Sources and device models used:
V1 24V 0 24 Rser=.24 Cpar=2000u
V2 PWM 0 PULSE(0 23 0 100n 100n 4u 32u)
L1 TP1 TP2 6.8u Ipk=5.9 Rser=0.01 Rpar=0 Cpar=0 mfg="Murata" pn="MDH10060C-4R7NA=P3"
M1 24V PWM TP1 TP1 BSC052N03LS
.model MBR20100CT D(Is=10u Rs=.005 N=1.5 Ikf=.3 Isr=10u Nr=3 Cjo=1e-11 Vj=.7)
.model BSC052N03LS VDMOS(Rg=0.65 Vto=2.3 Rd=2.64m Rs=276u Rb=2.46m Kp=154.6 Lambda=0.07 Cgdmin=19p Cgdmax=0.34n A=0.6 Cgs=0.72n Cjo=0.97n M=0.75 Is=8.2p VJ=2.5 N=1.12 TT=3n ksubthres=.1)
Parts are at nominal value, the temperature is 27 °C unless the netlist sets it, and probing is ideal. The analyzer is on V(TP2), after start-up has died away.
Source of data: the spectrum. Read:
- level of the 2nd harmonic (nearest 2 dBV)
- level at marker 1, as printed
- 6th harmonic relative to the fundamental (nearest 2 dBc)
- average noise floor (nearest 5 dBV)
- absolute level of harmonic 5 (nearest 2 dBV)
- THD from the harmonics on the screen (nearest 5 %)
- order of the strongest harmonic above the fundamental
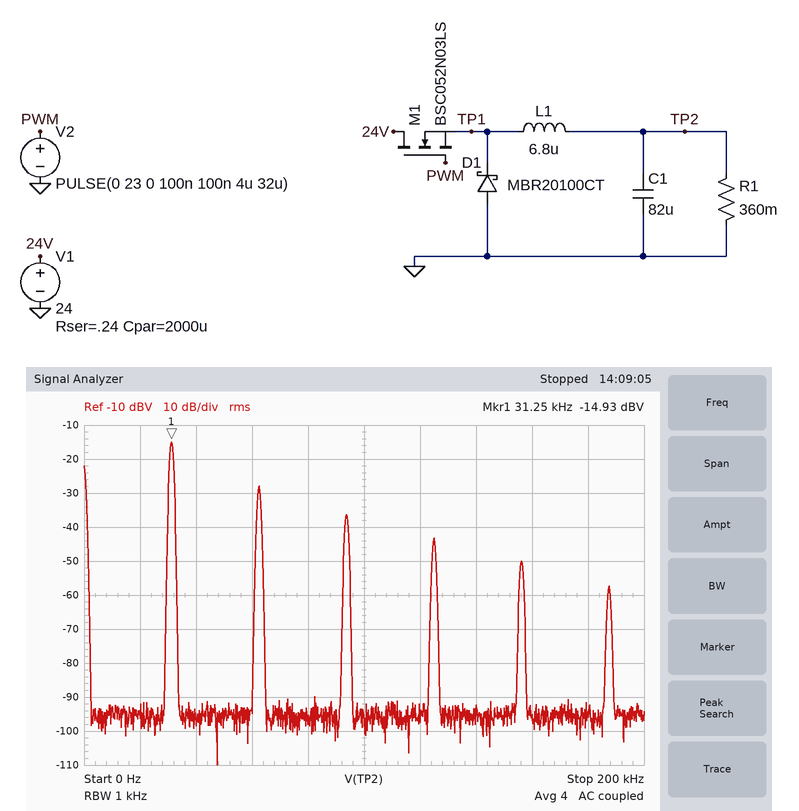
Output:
-28 dBV
-14.93 dBV
-42 dBc
-95 dBV
-50 dBV
25 %
2
